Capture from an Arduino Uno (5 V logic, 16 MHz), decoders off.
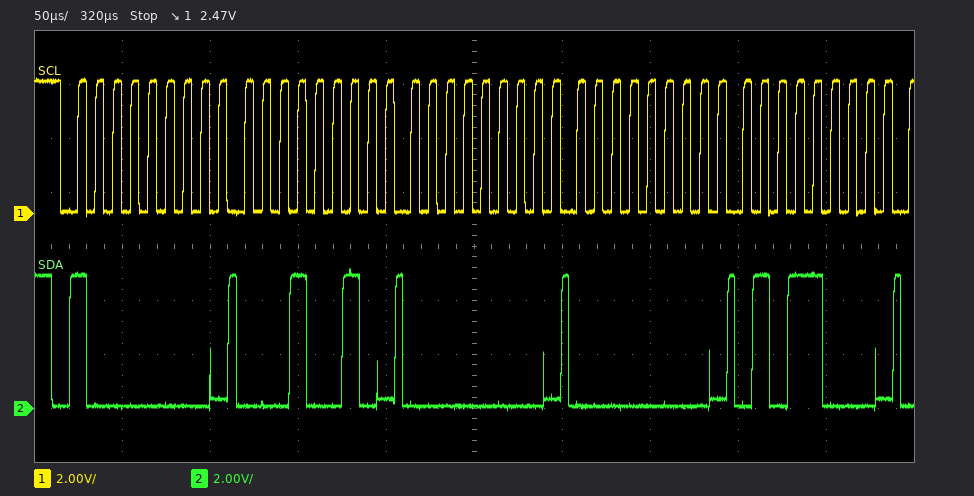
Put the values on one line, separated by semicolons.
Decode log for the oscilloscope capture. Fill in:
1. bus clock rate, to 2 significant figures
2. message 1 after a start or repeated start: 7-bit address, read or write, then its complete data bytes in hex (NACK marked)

100 kHz; 0x40 write: 12 00 00 58
